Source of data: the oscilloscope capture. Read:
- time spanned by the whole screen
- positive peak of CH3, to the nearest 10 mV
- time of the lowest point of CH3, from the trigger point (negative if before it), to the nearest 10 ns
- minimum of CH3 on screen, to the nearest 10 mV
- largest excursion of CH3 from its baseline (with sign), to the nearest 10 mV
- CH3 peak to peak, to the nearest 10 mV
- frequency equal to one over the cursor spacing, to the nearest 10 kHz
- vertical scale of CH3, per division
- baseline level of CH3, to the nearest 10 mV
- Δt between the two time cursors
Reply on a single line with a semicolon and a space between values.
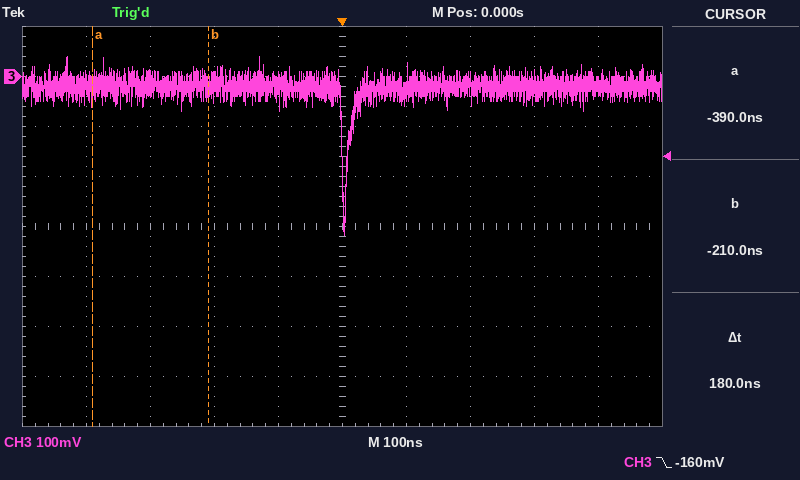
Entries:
1 µs; 40 mV; 0 ns; -320 mV; -300 mV; 360 mV; 5.56 MHz; 100 mV; -20 mV; 180 ns
